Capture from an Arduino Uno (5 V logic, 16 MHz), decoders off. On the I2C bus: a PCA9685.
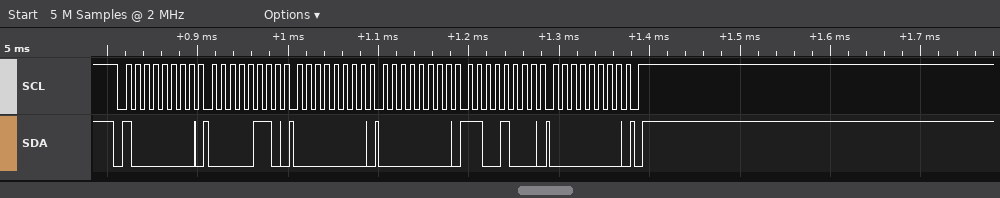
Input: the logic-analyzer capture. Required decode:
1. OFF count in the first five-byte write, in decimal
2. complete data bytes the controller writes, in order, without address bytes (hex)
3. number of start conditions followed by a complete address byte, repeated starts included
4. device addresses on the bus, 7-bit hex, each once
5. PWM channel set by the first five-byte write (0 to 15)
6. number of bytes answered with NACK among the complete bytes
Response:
200
06 00 00 C8 00
1
0x40
0
0
